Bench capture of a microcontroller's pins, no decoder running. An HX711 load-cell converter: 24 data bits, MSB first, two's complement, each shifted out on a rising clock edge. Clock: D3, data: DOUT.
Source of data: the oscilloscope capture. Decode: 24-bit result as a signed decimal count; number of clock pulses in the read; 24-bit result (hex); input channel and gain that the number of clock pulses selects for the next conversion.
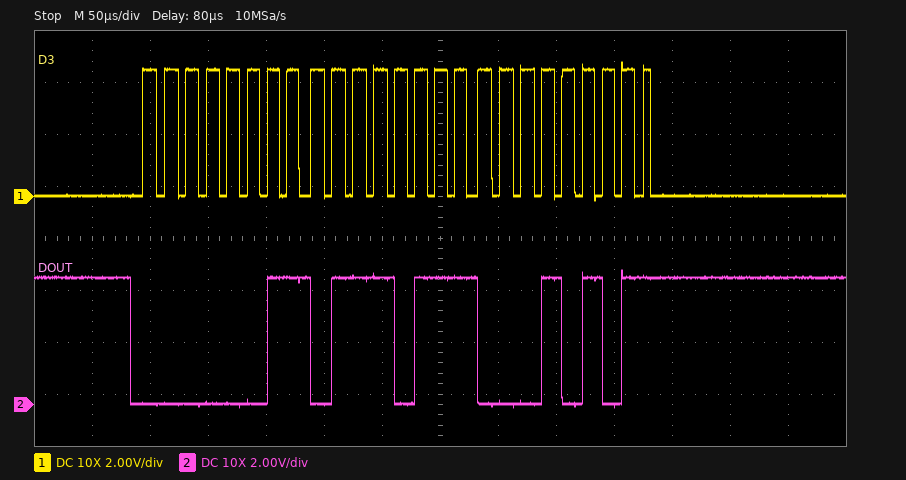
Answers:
227093
25
0x037715
channel A, gain 128
